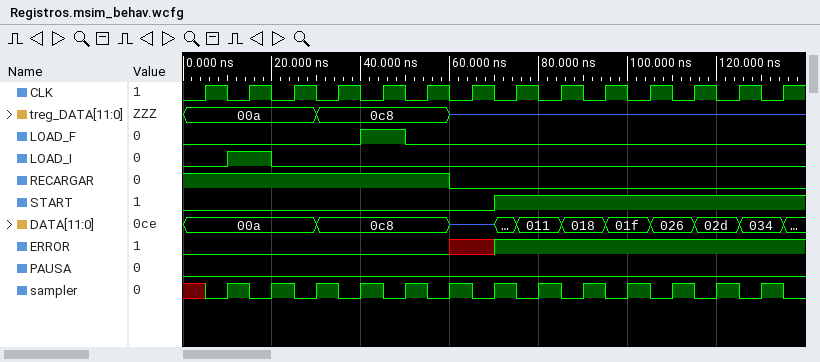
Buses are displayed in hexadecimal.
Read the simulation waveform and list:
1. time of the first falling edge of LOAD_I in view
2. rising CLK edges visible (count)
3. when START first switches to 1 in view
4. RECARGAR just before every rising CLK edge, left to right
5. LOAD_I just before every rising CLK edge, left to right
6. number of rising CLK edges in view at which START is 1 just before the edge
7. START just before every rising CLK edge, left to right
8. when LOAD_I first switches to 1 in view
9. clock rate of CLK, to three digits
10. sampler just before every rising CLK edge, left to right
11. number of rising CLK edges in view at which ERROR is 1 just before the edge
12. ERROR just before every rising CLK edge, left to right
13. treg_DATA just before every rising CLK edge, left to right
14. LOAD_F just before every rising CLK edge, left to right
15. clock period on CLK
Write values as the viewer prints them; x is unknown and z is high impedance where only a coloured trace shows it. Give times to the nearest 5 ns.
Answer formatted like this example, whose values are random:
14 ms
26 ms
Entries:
20 ns
14
70 ns
1 1 1 1 1 1 0 0 0 0 0 0 0 0
0 1 0 0 0 0 0 0 0 0 0 0 0 0
7
0 0 0 0 0 0 0 1 1 1 1 1 1 1
10 ns
100 MHz
x 1 1 1 1 1 1 1 1 1 1 1 1 1
7
0 0 0 0 0 0 x 1 1 1 1 1 1 1
00a, 00a, 00a, 0c8, 0c8, 0c8, z, z, z, z, z, z, z, z
0 0 0 0 1 0 0 0 0 0 0 0 0 0
10 ns
